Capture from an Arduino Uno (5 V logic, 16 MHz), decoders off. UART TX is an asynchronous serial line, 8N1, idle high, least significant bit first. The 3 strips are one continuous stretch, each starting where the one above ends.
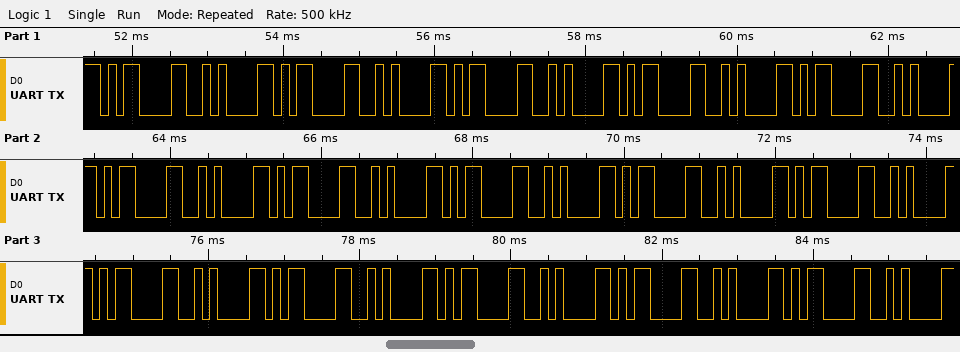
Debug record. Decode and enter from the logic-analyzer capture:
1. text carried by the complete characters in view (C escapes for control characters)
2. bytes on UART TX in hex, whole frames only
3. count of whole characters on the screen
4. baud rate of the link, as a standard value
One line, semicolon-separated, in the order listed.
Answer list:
"\r\n\r\n\r\n\r\n\r\n\r\n\r\n\r\n\r\n\r\n\r\n\r\n\r\n\r\n\r\n"; 0D 0A 0D 0A 0D 0A 0D 0A 0D 0A 0D 0A 0D 0A 0D 0A 0D 0A 0D 0A 0D 0A 0D 0A 0D 0A 0D 0A 0D 0A; 30; 9600 baud
